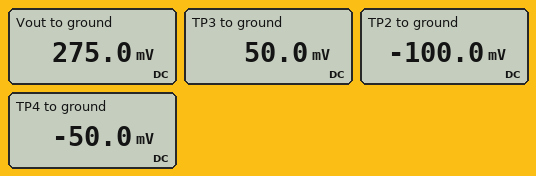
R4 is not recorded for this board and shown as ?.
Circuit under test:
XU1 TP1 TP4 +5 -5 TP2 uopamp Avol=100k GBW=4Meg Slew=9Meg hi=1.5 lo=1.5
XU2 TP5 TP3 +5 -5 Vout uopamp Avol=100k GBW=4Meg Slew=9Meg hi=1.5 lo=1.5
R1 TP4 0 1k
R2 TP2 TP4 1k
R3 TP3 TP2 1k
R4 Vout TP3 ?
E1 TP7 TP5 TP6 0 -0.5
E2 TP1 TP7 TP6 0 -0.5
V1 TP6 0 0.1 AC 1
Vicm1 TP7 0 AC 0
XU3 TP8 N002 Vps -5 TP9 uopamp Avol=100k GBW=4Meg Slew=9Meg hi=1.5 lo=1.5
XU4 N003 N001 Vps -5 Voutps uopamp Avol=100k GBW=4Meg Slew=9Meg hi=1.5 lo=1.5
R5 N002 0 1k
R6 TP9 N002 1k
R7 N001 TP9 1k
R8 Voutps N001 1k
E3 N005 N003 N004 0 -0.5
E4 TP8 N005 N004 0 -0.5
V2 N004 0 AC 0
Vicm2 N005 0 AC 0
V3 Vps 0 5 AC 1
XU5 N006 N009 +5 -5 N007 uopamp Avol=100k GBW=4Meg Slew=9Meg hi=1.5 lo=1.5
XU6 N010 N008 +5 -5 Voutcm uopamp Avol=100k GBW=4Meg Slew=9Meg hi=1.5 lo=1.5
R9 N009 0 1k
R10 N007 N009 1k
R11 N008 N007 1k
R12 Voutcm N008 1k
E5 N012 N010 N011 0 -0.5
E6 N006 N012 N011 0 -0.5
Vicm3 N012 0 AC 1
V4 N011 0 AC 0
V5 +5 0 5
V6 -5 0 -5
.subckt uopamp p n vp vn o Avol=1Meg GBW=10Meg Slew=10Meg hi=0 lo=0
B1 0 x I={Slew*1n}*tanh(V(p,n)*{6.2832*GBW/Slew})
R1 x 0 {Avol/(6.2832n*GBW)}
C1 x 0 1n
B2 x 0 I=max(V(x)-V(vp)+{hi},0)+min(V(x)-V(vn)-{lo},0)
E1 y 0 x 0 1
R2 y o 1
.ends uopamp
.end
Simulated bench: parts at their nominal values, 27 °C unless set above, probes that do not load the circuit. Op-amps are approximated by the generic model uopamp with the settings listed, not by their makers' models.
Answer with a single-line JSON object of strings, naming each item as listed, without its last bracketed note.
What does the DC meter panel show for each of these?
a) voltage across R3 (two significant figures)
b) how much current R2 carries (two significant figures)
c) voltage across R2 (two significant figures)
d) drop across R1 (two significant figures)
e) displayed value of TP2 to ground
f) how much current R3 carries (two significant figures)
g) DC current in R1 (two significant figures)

{"voltage across R3": "150 mV", "how much current R2 carries": "50 µA", "voltage across R2": "50 mV", "drop across R1": "50 mV", "displayed value of TP2 to ground": "-100.0 mV", "how much current R3 carries": "150 µA", "DC current in R1": "50 µA"}
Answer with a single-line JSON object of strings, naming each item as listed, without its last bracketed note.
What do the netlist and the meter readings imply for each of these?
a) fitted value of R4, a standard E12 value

{"fitted value of R4, a standard E12 value": "1.5 kΩ"}
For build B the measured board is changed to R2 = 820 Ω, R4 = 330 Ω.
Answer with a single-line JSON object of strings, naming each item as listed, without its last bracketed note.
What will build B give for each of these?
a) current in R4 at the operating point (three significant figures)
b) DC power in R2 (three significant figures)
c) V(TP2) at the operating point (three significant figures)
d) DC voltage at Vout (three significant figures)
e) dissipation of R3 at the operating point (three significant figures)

{"current in R4 at the operating point": "141 µA", "DC power in R2": "2.05 µW", "V(TP2) at the operating point": "-91.0 mV", "DC voltage at Vout": "96.5 mV", "dissipation of R3 at the operating point": "19.9 µW"}
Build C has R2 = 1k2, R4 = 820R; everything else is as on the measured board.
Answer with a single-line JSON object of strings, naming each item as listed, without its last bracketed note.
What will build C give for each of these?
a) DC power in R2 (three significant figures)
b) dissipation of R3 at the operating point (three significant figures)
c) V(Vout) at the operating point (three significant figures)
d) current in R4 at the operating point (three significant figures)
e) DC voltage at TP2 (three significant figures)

{"DC power in R2": "3.00 µW", "dissipation of R3 at the operating point": "25.6 µW", "V(Vout) at the operating point": "181 mV", "current in R4 at the operating point": "160 µA", "DC voltage at TP2": "-110 mV"}
